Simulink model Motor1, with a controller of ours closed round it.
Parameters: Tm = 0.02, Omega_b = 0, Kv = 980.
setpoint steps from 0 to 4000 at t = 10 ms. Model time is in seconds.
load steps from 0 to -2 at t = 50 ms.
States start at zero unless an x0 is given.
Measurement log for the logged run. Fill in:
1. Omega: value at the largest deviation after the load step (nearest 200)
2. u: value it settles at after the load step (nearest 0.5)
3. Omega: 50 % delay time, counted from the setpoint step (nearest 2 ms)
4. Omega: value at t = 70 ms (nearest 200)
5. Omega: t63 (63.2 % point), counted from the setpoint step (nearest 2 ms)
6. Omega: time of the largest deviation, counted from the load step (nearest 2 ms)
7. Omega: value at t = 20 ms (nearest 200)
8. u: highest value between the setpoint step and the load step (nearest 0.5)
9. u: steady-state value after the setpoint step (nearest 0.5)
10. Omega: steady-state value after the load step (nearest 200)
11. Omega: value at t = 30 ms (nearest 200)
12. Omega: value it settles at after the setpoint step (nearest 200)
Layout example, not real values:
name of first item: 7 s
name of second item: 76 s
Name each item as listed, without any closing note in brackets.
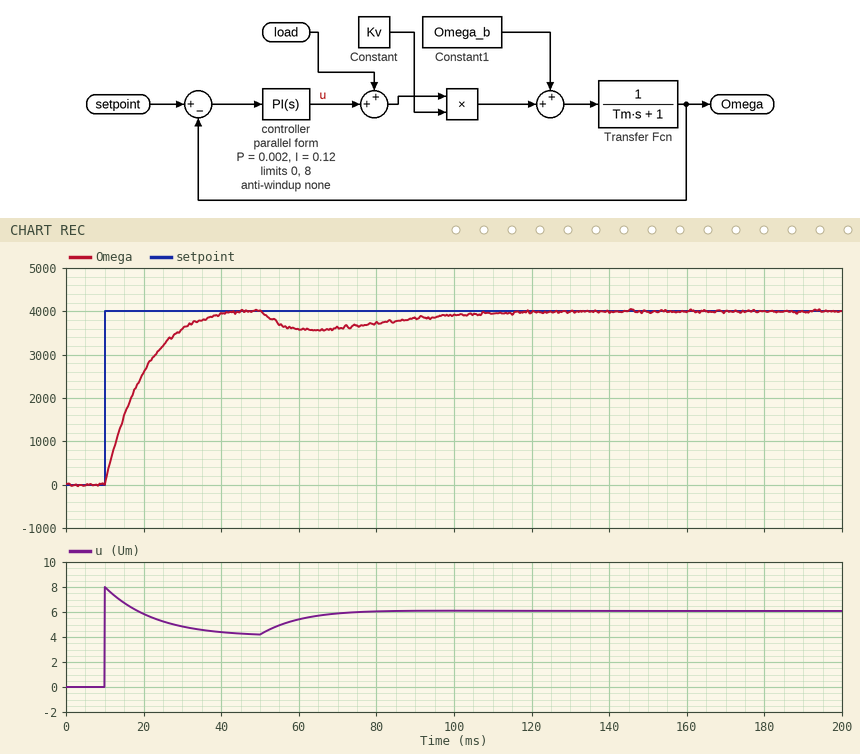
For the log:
Omega: value at the largest deviation after the load step: 3600
u: value it settles at after the load step: 6.0
Omega: 50 % delay time, counted from the setpoint step: 6 ms
Omega: value at t = 70 ms: 3600
Omega: t63 (63.2 % point), counted from the setpoint step: 10 ms
Omega: time of the largest deviation, counted from the load step: 14 ms
Omega: value at t = 20 ms: 2600
u: highest value between the setpoint step and the load step: 8.0
u: steady-state value after the setpoint step: 4.0
Omega: steady-state value after the load step: 4000
Omega: value at t = 30 ms: 3600
Omega: value it settles at after the setpoint step: 4000
